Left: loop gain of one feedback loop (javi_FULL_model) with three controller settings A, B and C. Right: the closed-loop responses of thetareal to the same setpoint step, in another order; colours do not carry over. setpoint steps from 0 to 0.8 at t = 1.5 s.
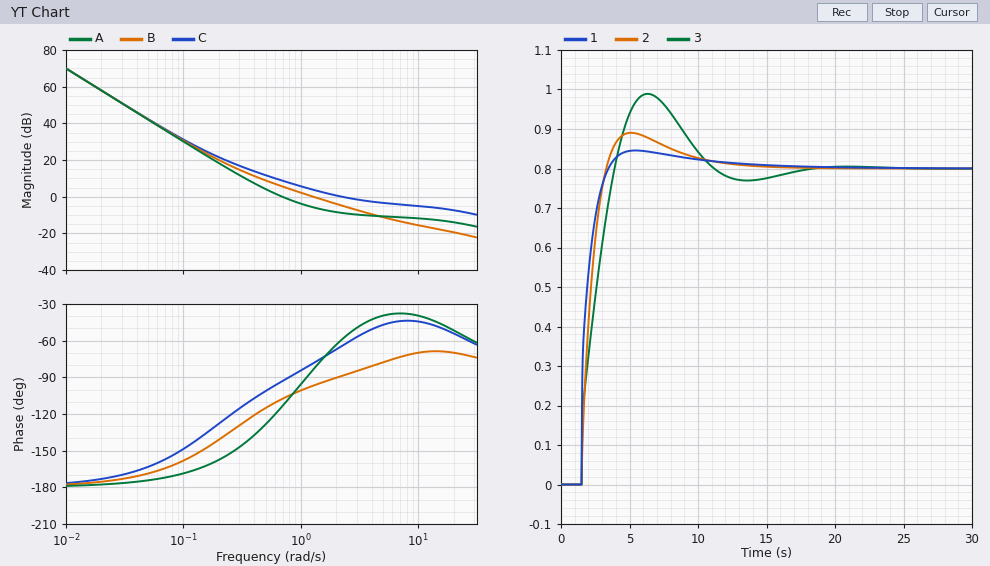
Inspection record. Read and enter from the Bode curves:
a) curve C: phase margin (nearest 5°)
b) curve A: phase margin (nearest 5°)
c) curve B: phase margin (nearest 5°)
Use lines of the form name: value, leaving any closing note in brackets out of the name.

curve C: phase margin: 115°
curve A: phase margin: 65°
curve B: phase margin: 85°
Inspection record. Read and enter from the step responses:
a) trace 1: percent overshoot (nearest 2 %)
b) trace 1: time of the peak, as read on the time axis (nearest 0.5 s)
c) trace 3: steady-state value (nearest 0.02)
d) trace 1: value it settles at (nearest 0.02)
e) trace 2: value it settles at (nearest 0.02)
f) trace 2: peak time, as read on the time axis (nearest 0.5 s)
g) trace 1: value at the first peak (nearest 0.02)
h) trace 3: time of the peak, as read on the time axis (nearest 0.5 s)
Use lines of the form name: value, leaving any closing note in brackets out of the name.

trace 1: percent overshoot: 6 %
trace 1: time of the peak, as read on the time axis: 5.5 s
trace 3: steady-state value: 0.80
trace 1: value it settles at: 0.80
trace 2: value it settles at: 0.80
trace 2: peak time, as read on the time axis: 5.0 s
trace 1: value at the first peak: 0.84
trace 3: time of the peak, as read on the time axis: 6.5 s
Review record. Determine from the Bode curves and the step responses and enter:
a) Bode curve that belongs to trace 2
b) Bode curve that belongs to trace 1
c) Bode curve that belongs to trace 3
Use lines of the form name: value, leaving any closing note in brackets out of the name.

Bode curve that belongs to trace 2: B
Bode curve that belongs to trace 1: C
Bode curve that belongs to trace 3: A
